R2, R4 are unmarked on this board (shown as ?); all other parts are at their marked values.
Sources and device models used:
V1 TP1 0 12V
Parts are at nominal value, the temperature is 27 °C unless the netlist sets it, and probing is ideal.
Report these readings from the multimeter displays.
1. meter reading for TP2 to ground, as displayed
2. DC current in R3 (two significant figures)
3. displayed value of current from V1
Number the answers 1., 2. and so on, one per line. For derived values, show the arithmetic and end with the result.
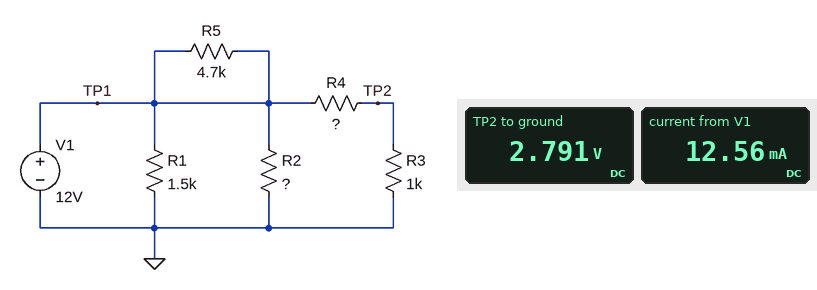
1. 2.791 V
2. (2.791 V) / 1 kΩ = 2.8 mA
3. 12.56 mA
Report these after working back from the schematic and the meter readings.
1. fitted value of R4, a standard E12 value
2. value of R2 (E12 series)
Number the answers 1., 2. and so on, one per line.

1. 3.3 kΩ
2. 6.8 kΩ
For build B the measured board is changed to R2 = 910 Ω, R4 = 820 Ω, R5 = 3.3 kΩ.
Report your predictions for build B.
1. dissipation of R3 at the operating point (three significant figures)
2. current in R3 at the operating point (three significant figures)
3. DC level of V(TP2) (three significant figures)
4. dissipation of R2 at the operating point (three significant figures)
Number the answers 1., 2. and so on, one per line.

1. 43.5 mW
2. 6.59 mA
3. 6.59 V
4. 158 mW
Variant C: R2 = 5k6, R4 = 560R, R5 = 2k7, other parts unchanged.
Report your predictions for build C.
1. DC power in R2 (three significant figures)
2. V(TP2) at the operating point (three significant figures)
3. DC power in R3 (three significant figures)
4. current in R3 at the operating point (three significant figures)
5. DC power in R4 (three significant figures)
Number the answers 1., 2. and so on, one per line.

1. 25.7 mW
2. 7.69 V
3. 59.2 mW
4. 7.69 mA
5. 33.1 mW
